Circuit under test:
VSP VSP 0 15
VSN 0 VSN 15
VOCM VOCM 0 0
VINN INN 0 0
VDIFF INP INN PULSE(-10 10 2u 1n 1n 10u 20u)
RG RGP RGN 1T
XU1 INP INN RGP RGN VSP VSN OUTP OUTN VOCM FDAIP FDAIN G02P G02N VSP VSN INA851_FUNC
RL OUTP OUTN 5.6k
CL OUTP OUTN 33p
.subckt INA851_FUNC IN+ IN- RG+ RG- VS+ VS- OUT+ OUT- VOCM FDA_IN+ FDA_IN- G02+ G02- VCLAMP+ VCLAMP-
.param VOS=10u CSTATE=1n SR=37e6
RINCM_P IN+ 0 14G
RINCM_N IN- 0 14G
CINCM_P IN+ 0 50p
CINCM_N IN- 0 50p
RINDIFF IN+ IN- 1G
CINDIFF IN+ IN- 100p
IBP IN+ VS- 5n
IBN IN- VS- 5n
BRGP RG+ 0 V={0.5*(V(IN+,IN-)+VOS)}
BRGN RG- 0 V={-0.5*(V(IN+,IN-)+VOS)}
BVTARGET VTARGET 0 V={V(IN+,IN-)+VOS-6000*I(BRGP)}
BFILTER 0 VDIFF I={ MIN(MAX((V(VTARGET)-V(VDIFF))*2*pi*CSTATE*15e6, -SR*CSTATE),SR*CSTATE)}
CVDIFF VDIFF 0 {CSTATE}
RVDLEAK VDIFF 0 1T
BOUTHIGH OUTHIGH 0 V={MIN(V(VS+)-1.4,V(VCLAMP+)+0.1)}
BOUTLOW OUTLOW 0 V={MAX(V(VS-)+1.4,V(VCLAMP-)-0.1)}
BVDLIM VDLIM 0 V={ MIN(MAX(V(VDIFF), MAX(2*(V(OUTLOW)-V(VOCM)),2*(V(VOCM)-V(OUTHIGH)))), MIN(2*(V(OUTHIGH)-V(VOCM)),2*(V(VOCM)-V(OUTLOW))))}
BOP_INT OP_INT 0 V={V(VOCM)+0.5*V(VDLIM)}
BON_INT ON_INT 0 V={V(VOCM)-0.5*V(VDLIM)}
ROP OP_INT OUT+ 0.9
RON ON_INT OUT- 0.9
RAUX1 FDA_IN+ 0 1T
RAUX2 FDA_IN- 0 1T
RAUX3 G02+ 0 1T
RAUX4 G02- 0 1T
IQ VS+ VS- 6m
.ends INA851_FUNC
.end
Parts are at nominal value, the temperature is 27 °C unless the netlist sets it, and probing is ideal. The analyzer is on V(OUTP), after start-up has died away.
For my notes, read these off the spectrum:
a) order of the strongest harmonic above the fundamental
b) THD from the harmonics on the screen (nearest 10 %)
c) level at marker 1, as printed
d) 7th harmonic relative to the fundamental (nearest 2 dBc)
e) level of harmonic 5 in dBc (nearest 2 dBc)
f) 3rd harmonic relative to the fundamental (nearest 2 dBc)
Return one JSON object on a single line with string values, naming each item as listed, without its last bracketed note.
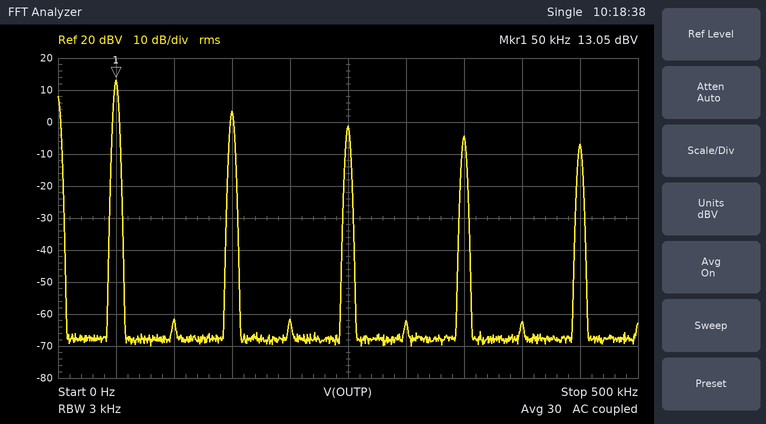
{"order of the strongest harmonic above the fundamental": "3", "THD from the harmonics on the screen": "40 %", "level at marker 1, as printed": "13.05 dBV", "7th harmonic relative to the fundamental": "-18 dBc", "level of harmonic 5 in dBc": "-14 dBc", "3rd harmonic relative to the fundamental": "-10 dBc"}
